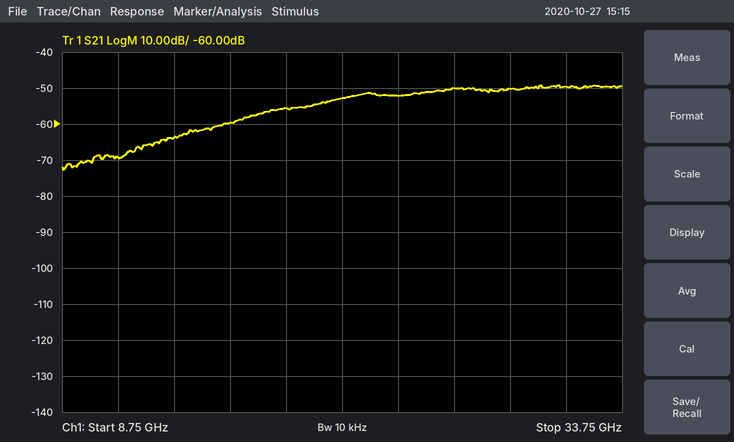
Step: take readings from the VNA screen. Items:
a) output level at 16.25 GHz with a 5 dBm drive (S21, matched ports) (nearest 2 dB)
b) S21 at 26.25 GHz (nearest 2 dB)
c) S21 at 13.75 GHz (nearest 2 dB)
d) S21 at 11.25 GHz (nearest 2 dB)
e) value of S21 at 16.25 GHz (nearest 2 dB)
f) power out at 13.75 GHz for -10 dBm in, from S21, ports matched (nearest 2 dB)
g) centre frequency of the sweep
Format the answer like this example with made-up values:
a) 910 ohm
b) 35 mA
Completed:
a) -54 dBm
b) -50 dB
c) -64 dB
d) -70 dB
e) -60 dB
f) -74 dBm
g) 21.25 GHz
